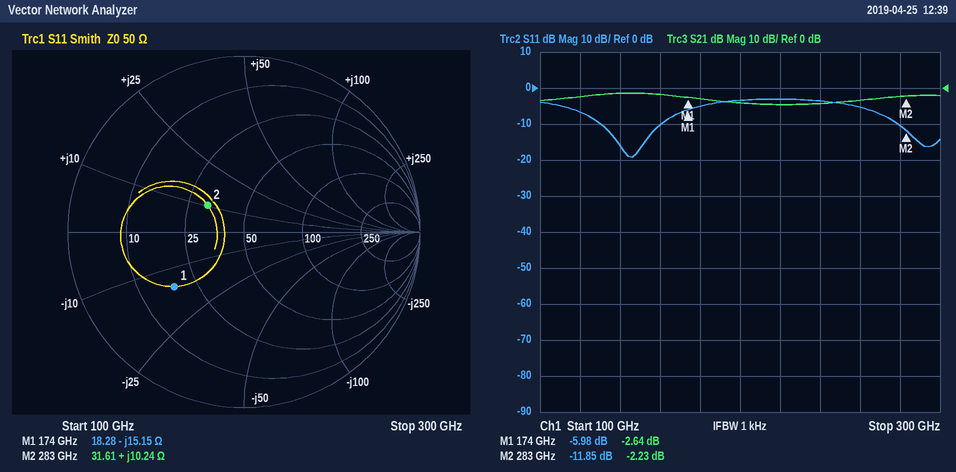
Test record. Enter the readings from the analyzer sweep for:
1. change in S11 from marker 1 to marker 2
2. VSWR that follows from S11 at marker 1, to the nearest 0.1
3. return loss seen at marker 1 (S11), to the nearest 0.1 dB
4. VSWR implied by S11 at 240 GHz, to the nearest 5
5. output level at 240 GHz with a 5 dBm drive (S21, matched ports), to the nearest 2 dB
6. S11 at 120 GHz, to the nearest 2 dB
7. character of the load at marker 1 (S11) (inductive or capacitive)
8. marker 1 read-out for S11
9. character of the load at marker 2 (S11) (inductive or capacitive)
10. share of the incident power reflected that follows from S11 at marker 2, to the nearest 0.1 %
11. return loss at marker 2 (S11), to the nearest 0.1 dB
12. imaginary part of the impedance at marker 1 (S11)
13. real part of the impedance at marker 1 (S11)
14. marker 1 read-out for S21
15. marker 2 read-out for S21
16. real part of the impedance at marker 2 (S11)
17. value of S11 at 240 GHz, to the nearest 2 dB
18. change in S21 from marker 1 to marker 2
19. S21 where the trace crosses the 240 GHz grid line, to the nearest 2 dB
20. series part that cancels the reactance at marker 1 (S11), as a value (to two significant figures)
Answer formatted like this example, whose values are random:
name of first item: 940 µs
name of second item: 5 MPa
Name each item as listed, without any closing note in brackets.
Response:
change in S11 from marker 1 to marker 2: -5.87 dB
VSWR that follows from S11 at marker 1, to the nearest 0.1: 3.0
return loss seen at marker 1 (S11), to the nearest 0.1 dB: 6.0 dB
VSWR implied by S11 at 240 GHz, to the nearest 5: 5
output level at 240 GHz with a 5 dBm drive (S21, matched ports), to the nearest 2 dB: 0 dBm
S11 at 120 GHz, to the nearest 2 dB: -6 dB
character of the load at marker 1 (S11): capacitive
marker 1 read-out for S11: -5.98 dB
character of the load at marker 2 (S11): inductive
share of the incident power reflected that follows from S11 at marker 2, to the nearest 0.1 %: 6.5 %
return loss at marker 2 (S11), to the nearest 0.1 dB: 11.8 dB
imaginary part of the impedance at marker 1: -15.15 Ω
real part of the impedance at marker 1: 18.28 Ω
marker 1 read-out for S21: -2.64 dB
marker 2 read-out for S21: -2.23 dB
real part of the impedance at marker 2: 31.61 Ω
value of S11 at 240 GHz, to the nearest 2 dB: -4 dB
change in S21 from marker 1 to marker 2: 0.41 dB
S21 where the trace crosses the 240 GHz grid line, to the nearest 2 dB: -4 dB
series part that cancels the reactance at marker 1 (S11), as a value: 14 pH
